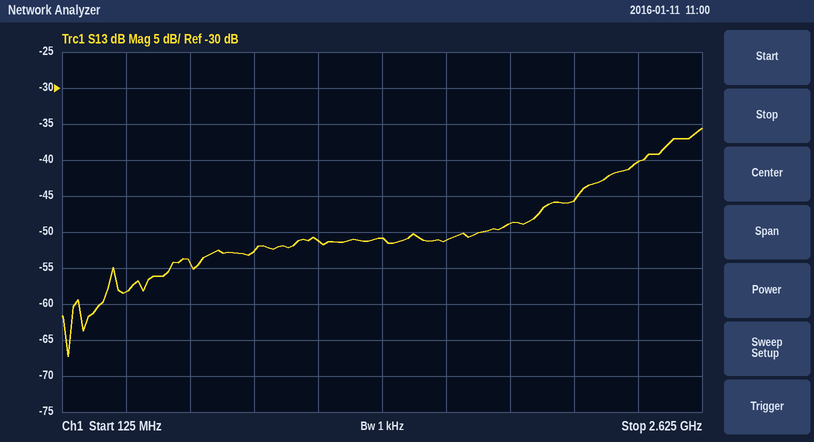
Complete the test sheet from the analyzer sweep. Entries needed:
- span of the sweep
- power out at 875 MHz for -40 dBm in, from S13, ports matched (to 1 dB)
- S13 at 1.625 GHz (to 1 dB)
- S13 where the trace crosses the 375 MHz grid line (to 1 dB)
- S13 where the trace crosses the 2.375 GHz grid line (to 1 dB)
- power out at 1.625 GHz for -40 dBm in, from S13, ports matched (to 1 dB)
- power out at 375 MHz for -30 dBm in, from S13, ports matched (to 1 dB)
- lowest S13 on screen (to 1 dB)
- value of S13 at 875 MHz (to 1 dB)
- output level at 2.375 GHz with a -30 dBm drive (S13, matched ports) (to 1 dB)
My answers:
2.5 GHz
-93 dBm
-51 dB
-58 dB
-40 dB
-91 dBm
-88 dBm
-67 dB
-53 dB
-70 dBm
